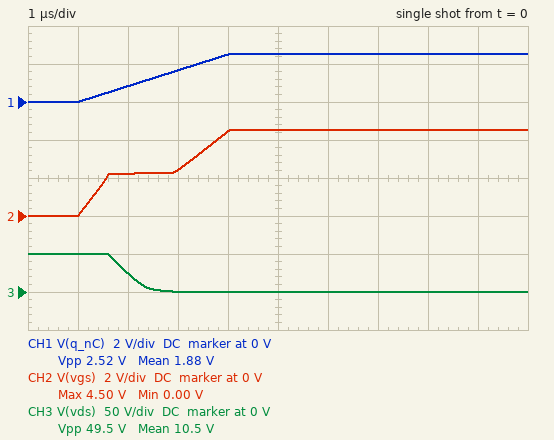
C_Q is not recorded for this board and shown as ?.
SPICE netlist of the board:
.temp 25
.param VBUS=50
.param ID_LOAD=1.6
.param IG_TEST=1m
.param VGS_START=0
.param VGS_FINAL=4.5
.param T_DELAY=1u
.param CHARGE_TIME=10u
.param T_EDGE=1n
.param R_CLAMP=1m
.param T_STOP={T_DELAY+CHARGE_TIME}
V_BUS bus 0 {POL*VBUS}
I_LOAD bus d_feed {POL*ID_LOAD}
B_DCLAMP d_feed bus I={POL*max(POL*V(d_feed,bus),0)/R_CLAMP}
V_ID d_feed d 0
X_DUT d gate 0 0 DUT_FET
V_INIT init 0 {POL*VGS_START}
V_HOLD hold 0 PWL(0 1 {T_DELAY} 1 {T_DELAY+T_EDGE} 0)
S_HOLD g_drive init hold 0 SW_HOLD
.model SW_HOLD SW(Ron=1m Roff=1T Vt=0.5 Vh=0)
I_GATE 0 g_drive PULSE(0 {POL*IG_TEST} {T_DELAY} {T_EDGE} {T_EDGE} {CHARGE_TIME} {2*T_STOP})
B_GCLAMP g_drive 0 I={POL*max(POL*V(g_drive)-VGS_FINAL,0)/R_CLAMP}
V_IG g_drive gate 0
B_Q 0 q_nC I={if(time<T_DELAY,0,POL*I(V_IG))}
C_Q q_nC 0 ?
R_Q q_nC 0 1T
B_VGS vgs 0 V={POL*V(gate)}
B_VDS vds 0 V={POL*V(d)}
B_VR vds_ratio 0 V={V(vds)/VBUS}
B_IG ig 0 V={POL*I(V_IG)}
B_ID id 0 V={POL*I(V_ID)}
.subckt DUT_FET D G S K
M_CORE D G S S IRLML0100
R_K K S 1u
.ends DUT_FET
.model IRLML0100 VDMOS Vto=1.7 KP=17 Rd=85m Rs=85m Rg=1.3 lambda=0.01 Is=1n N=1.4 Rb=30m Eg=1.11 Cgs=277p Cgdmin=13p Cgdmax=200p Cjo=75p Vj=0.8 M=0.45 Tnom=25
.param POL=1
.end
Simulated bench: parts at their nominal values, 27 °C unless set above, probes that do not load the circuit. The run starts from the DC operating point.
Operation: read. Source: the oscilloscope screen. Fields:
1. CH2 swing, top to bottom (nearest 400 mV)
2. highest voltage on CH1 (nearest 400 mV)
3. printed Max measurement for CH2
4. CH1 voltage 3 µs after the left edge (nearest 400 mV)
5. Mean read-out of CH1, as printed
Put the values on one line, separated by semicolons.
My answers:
4.4 V; 2.4 V; 4.50 V; 1.6 V; 1.88 V
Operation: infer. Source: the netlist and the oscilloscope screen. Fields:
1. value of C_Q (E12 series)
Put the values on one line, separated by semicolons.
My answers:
1.2 nF
